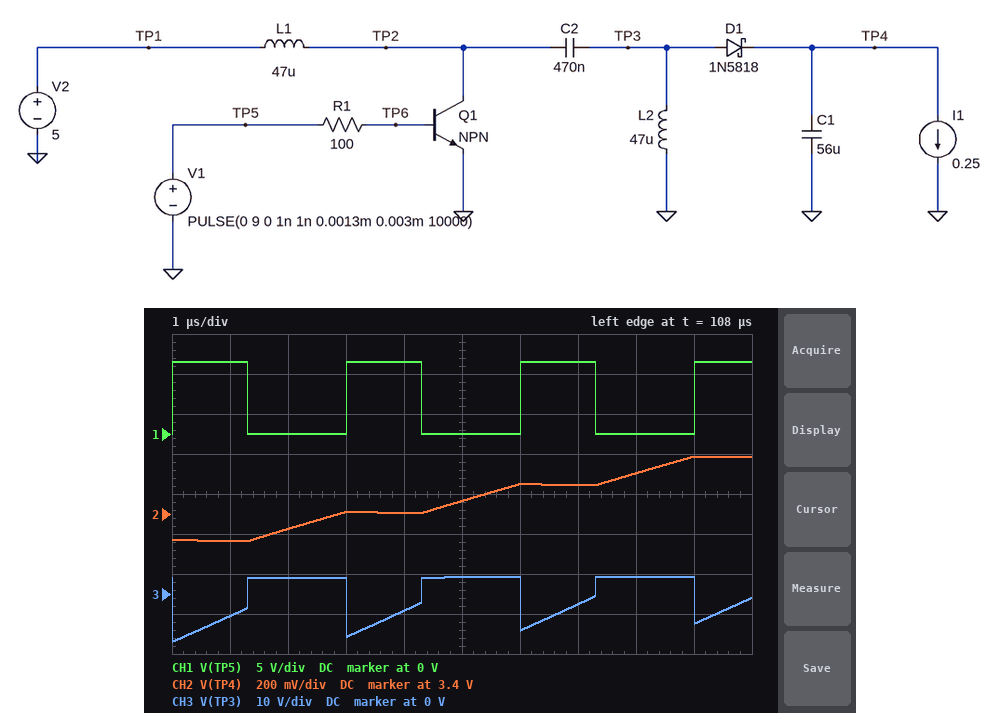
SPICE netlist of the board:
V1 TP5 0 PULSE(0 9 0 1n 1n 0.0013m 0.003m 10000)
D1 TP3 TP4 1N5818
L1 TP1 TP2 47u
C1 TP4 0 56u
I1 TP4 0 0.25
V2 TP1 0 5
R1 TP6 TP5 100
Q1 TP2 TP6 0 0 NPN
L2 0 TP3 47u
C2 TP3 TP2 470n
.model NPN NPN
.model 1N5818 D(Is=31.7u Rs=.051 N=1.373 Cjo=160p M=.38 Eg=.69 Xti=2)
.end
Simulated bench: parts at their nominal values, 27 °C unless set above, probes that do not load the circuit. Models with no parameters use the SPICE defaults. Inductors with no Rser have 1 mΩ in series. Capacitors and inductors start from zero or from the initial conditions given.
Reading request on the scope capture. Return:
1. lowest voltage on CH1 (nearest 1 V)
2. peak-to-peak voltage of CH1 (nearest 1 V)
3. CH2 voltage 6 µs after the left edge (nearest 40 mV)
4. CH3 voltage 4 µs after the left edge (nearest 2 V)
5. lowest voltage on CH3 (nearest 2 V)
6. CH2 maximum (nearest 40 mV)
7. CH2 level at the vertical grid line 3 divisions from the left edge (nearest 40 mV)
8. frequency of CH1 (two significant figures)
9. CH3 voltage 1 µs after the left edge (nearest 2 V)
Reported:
0 V
9 V
3.56 V
-4 V
-12 V
3.68 V
3.40 V
330 kHz
-6 V
